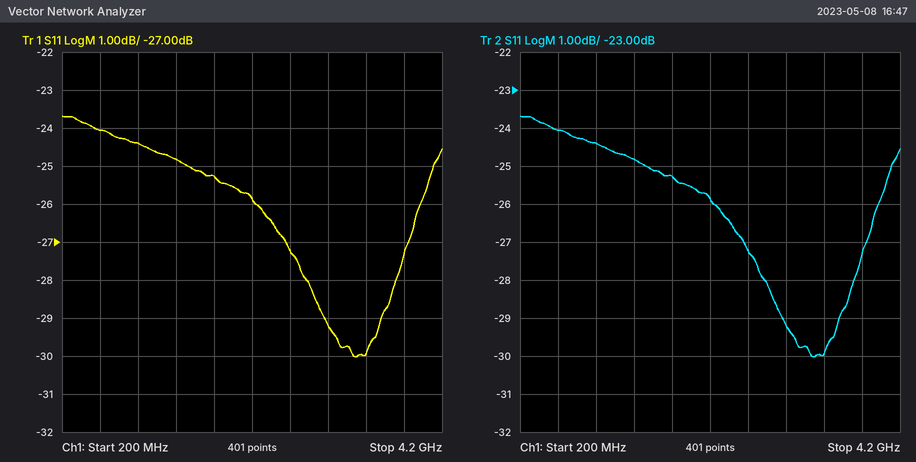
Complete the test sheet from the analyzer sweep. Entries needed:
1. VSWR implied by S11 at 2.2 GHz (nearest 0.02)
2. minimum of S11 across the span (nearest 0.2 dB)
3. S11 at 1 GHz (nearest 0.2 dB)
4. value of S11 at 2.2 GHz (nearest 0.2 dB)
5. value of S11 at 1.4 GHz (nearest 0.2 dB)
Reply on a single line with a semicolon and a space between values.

1.10; -30.0 dB; -24.4 dB; -25.8 dB; -24.8 dB
